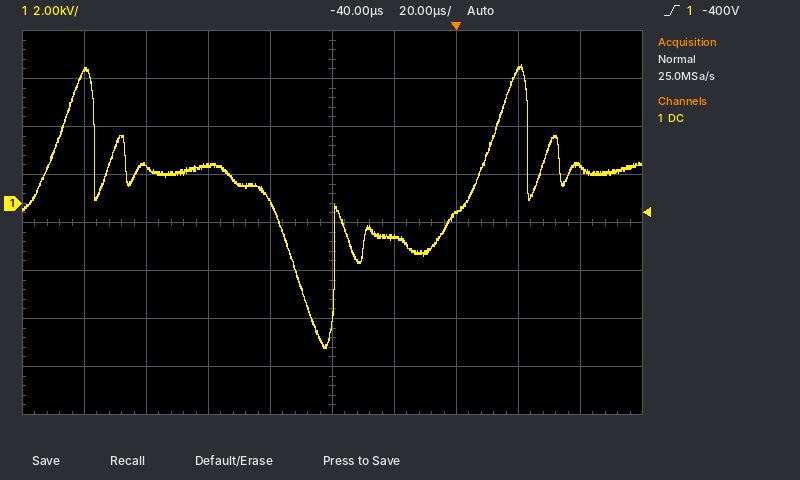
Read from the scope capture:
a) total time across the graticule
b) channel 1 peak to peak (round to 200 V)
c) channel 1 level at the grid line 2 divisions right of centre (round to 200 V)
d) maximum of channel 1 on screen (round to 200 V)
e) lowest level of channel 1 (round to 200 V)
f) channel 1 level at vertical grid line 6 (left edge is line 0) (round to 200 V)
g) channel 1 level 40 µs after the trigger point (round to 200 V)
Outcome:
200 µs
11.8 kV
-400 V
5.8 kV
-6.0 kV
-1.4 kV
1.6 kV
